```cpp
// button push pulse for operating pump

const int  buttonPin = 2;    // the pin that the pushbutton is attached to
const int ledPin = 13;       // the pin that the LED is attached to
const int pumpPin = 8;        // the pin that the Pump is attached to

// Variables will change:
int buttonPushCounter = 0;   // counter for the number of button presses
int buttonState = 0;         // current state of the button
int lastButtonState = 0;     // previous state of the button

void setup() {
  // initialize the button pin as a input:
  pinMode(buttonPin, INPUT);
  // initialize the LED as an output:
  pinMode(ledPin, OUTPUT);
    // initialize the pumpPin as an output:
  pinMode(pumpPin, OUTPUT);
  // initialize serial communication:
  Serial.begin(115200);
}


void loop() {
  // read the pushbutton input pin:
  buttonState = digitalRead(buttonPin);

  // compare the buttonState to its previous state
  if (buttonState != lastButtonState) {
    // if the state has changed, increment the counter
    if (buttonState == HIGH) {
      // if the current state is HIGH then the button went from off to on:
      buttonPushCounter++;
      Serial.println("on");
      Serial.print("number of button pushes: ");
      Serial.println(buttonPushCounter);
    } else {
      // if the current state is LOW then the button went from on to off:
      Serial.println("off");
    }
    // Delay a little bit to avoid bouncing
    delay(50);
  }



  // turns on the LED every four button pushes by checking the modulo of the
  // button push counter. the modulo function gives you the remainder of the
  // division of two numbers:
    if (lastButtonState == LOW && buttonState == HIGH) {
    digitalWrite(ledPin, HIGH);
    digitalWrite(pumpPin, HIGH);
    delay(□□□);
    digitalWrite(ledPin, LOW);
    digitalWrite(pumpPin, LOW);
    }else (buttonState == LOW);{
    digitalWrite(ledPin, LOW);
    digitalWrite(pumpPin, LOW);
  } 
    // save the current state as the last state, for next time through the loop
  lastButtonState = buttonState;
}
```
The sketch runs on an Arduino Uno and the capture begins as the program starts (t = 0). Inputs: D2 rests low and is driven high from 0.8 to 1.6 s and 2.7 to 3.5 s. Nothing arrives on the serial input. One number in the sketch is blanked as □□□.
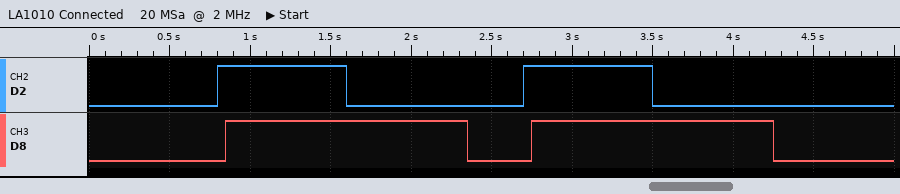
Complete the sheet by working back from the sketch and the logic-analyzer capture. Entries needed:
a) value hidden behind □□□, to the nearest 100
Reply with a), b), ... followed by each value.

a) 1500
